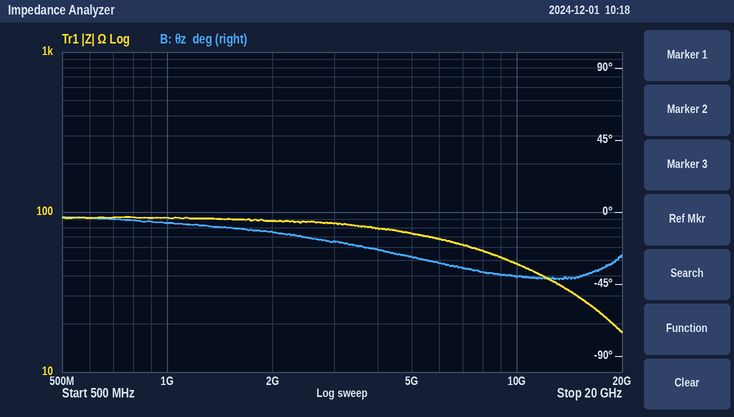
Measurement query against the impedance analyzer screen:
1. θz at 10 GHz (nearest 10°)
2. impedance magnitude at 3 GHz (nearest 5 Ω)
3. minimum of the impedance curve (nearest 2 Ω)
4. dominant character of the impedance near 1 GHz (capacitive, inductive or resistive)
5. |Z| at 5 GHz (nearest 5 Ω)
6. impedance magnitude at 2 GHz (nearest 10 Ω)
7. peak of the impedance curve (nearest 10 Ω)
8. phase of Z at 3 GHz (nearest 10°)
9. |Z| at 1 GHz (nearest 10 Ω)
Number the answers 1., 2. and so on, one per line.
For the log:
1. -40°
2. 85 Ω
3. 18 Ω
4. resistive
5. 75 Ω
6. 90 Ω
7. 90 Ω
8. -20°
9. 90 Ω
